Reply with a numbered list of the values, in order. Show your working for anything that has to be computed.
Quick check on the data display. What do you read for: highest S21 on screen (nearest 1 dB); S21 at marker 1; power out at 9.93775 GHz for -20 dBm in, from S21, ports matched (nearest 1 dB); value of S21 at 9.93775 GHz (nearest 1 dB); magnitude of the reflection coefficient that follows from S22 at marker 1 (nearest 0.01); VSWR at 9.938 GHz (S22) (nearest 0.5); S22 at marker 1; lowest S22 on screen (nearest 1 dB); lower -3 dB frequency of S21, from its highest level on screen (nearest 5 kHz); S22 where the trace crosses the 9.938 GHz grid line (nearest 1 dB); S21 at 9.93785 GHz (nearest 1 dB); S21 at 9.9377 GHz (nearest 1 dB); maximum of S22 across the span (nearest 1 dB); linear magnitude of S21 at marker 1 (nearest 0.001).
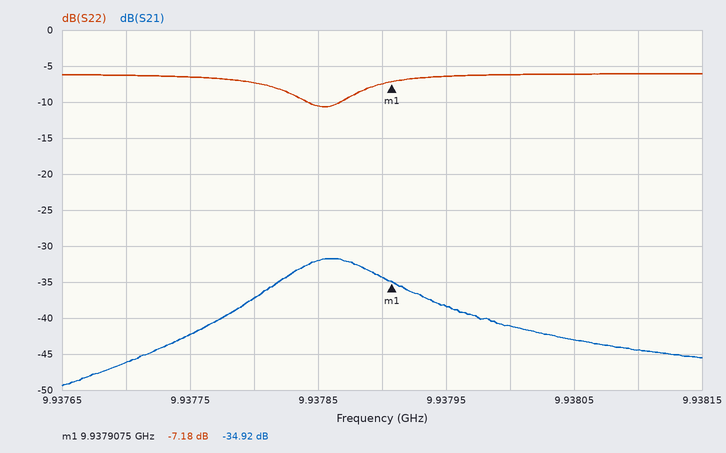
1. -32 dB
2. -34.92 dB
3. -20 dBm + (-42 dB) = -62 dBm
4. -42 dB
5. 10^(-7.18/20) ≈ 0.44
6. |Γ| = 10^(-6/20) = 0.5012; VSWR = (1 + 0.5012)/(1 − 0.5012) ≈ 3.0
7. -7.18 dB
8. -11 dB
9. 9.937820 GHz
10. -6 dB
11. -32 dB
12. -46 dB
13. -6 dB
14. 10^(-34.92/20) ≈ 0.018
